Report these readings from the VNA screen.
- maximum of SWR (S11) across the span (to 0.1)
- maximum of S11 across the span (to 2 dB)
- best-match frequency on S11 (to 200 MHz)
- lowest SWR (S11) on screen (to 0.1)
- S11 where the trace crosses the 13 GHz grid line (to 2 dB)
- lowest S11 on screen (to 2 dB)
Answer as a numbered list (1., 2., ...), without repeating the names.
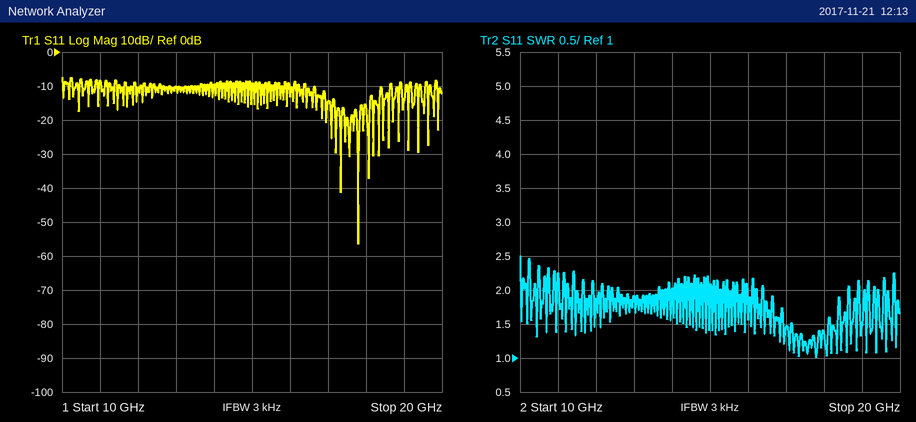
1. 2.5
2. -8 dB
3. 17.8 GHz
4. 1.0
5. -10 dB
6. -56 dB
